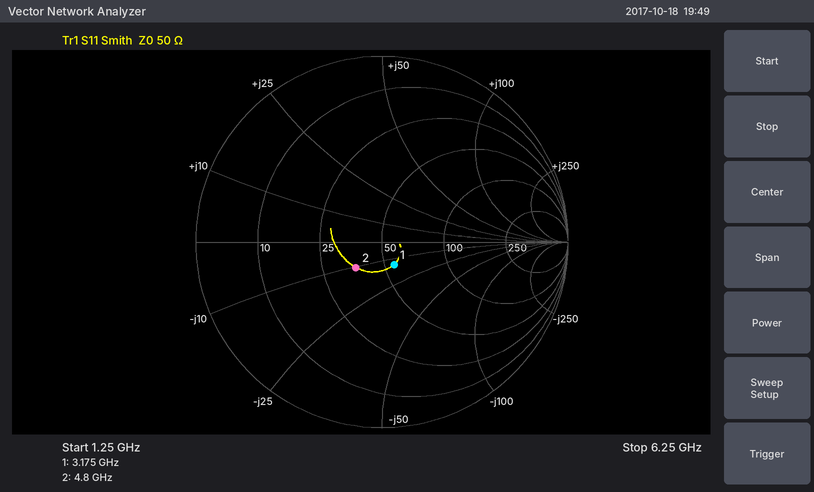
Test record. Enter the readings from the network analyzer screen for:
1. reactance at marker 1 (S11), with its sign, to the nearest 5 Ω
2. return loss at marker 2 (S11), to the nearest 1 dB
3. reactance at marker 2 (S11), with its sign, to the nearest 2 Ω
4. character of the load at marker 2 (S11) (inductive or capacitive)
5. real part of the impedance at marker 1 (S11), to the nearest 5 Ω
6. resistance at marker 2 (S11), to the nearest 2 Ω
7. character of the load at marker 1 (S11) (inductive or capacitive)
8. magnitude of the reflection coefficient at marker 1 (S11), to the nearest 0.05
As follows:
-15 Ω
14 dB
-10 Ω
capacitive
55 Ω
36 Ω
capacitive
0.15
